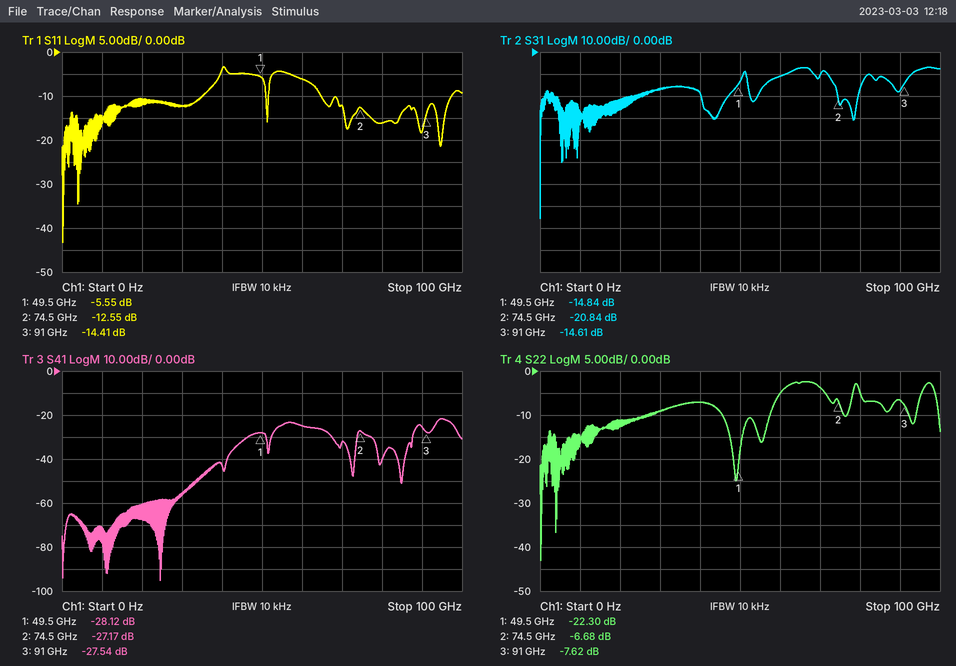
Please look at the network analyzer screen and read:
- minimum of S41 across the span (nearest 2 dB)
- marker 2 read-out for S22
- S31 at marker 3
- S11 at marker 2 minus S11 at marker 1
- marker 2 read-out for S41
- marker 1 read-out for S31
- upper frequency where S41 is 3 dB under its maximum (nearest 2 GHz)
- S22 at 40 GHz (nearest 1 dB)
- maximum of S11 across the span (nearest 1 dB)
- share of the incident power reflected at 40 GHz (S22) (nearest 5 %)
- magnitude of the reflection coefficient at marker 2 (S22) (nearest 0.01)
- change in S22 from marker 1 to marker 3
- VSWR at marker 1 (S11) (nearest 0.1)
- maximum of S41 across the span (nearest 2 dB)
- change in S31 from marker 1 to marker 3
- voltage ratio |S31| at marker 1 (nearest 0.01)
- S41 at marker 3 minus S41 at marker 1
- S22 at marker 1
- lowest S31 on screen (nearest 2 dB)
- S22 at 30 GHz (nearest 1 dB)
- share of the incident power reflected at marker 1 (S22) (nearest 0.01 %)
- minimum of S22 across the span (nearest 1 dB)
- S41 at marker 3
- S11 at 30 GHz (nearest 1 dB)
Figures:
-96 dB
-6.68 dB
-14.61 dB
-7.00 dB
-27.17 dB
-14.84 dB
98 GHz
-7 dB
-3 dB
20 %
0.46
14.68 dB
3.2
-22 dB
0.23 dB
0.18
0.58 dB
-22.30 dB
-76 dB
-9 dB
0.59 %
-43 dB
-27.54 dB
-12 dB
